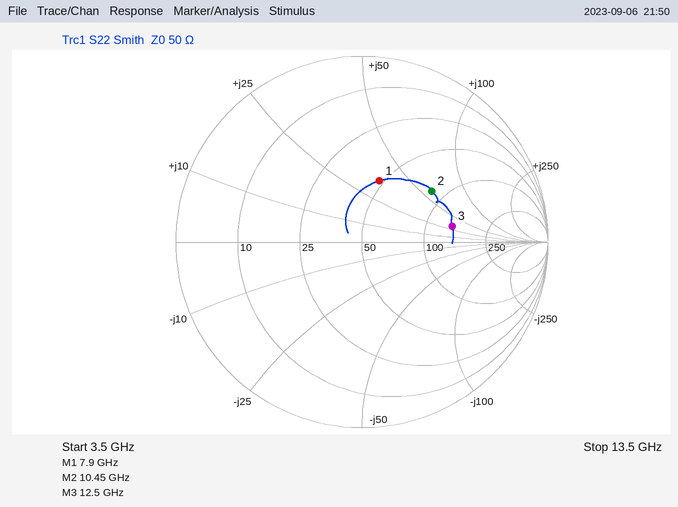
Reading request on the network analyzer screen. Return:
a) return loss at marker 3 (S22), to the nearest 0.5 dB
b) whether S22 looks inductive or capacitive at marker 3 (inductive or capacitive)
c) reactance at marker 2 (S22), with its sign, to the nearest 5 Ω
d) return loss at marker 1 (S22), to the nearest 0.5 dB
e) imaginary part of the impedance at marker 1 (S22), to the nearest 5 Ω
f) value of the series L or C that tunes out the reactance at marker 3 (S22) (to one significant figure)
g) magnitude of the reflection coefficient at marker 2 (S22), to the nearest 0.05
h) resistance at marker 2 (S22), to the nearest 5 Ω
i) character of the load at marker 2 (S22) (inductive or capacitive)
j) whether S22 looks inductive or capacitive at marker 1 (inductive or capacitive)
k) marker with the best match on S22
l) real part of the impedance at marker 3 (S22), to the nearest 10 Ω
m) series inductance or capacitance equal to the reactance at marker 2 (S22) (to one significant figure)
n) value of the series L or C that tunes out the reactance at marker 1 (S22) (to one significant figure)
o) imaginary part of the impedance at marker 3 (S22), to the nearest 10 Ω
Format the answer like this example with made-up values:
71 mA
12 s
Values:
6.0 dB
inductive
+60 Ω
9.5 dB
+35 Ω
400 fF
0.45
85 Ω
inductive
inductive
marker 1
140 Ω
900 pH
600 fF
+30 Ω
